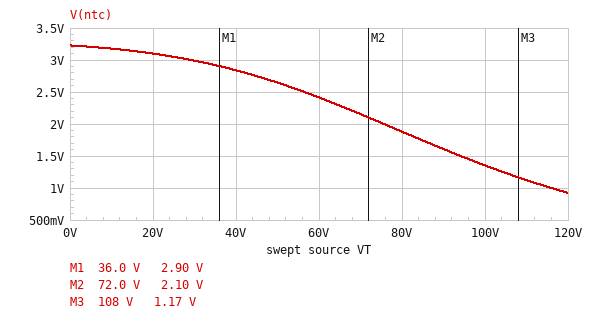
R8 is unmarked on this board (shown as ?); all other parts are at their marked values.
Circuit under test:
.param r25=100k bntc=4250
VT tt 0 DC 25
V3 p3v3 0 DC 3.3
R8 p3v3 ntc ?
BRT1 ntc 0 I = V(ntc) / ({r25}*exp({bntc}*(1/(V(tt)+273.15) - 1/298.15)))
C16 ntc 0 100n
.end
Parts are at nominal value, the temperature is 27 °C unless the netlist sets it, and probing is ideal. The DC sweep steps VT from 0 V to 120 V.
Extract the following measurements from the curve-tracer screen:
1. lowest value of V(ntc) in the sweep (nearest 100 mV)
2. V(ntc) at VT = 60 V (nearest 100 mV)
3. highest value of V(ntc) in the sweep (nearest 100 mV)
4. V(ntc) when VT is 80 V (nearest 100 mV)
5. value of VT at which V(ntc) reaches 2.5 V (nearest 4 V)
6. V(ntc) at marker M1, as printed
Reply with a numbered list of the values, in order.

1. 900 mV
2. 2.4 V
3. 3.2 V
4. 1.9 V
5. 56 V
6. 2.90 V
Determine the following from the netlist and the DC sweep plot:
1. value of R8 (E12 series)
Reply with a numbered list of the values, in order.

1. 8.2 kΩ
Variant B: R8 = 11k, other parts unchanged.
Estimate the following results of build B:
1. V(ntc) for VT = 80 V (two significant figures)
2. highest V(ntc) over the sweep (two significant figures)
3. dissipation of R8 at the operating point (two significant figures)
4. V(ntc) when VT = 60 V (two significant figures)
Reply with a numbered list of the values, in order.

1. 1.6 V
2. 3.2 V
3. 9.7 µW
4. 2.2 V
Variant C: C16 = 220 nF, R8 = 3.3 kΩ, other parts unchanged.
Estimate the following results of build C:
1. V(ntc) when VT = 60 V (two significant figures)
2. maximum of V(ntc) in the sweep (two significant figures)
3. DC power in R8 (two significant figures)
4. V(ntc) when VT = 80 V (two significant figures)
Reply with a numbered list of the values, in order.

1. 2.9 V
2. 3.3 V
3. 3.4 µW
4. 2.5 V
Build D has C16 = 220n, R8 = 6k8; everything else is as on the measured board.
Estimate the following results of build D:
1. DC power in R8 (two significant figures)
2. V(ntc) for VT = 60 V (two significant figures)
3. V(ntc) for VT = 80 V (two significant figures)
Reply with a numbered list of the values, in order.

1. 6.5 µW
2. 2.5 V
3. 2.0 V
